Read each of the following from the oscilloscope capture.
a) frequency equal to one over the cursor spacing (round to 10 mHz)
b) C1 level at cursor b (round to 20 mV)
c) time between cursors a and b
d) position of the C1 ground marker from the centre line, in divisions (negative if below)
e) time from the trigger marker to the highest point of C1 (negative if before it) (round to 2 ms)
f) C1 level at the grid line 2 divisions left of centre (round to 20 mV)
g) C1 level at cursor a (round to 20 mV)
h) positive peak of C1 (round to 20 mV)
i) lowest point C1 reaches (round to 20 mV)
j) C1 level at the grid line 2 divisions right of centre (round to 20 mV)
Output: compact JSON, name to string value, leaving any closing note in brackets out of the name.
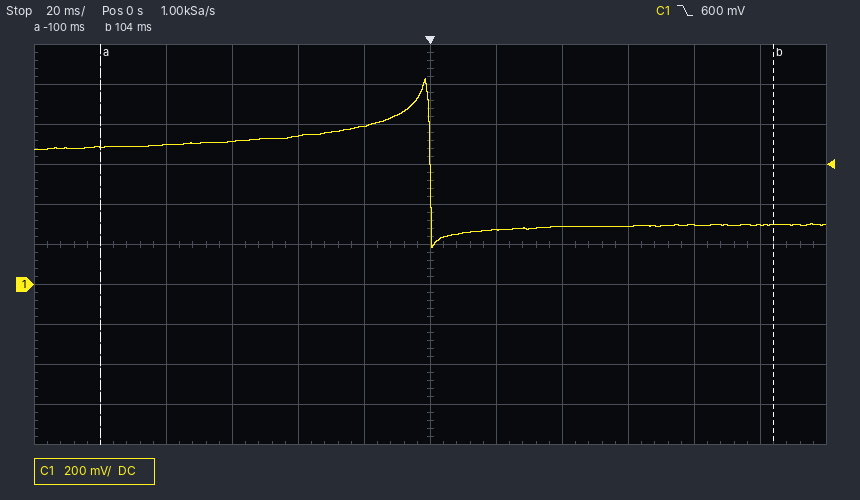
{"frequency equal to one over the cursor spacing": "4.90 Hz", "C1 level at cursor b": "300 mV", "time between cursors a and b": "204 ms", "position of the C1 ground marker from the centre line, in divisions": "-1.0 div", "time from the trigger marker to the highest point of C1 (negative if before it)": "-2 ms", "C1 level at the grid line 2 divisions left of centre": "740 mV", "C1 level at cursor a": "680 mV", "positive peak of C1": "1.04 V", "lowest point C1 reaches": "180 mV", "C1 level at the grid line 2 divisions right of centre": "280 mV"}
